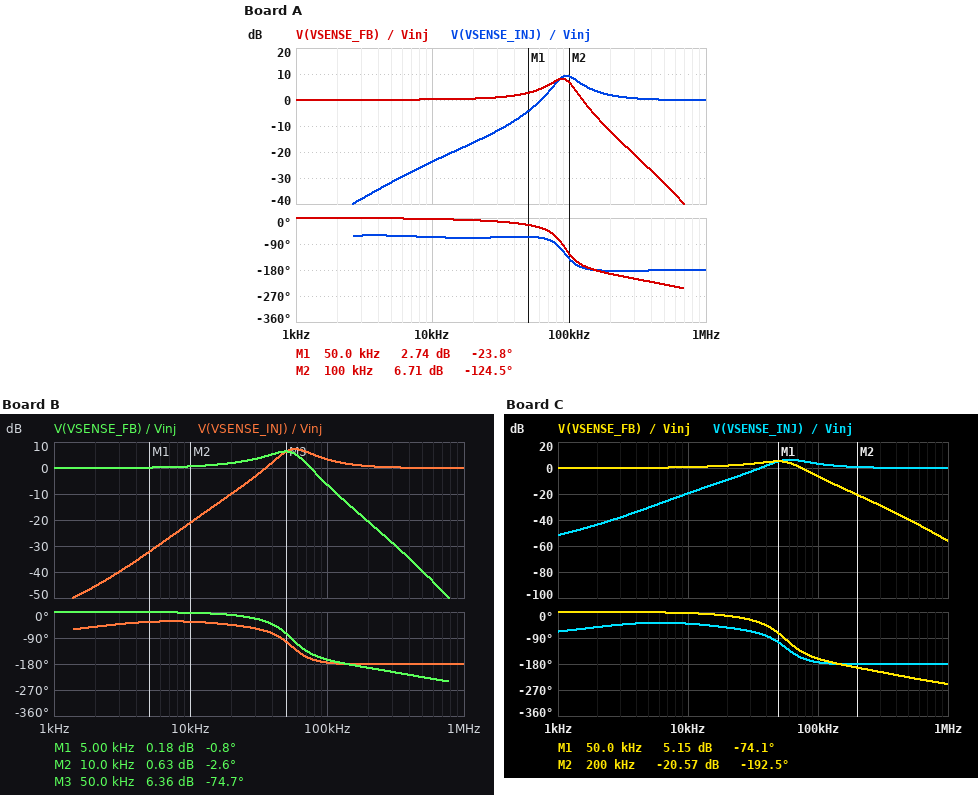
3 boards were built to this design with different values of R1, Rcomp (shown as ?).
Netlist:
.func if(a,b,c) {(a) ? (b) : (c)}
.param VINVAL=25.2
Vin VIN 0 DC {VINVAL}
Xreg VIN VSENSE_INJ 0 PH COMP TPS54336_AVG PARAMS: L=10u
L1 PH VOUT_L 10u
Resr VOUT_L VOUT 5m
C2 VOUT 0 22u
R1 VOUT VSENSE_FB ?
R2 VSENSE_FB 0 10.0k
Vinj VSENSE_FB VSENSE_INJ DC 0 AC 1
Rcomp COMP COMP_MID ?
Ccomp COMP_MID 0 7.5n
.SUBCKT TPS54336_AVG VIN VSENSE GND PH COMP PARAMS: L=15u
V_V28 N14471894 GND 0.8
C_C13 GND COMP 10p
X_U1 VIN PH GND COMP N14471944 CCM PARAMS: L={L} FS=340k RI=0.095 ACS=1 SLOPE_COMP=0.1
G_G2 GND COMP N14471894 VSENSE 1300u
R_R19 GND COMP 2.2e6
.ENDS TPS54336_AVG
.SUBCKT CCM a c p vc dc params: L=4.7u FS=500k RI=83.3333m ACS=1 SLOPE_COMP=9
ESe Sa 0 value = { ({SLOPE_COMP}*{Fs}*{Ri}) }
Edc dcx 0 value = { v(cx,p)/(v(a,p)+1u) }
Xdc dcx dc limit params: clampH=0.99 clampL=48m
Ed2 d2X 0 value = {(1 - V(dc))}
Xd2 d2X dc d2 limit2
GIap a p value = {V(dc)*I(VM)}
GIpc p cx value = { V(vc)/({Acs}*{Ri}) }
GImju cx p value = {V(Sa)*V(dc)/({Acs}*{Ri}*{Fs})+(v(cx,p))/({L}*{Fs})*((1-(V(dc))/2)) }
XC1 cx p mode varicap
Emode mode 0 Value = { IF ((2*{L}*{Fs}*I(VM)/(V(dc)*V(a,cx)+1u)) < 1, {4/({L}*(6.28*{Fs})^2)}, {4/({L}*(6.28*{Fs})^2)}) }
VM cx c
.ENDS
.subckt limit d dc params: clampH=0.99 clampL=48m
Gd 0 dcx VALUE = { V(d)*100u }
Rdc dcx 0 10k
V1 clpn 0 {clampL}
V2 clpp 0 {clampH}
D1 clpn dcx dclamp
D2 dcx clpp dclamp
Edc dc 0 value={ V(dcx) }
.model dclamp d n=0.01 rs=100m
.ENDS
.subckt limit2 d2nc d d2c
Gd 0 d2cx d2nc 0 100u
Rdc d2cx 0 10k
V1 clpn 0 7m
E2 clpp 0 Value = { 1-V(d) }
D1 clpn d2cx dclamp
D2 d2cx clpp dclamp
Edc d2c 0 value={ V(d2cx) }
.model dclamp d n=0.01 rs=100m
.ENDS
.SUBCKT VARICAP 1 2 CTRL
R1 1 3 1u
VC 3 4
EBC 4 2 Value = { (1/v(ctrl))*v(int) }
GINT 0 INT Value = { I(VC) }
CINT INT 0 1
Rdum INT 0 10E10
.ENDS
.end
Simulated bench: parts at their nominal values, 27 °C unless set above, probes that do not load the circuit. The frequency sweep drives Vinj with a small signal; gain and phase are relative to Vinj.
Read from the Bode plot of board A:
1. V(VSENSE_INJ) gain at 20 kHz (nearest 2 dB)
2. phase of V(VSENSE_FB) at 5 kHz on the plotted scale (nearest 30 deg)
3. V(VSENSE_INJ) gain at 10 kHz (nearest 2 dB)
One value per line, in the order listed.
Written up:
-16 dB
0 deg
-24 dB
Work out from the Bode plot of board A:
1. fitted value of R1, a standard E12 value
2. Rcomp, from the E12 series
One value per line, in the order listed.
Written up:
18 kΩ
3.9 kΩ
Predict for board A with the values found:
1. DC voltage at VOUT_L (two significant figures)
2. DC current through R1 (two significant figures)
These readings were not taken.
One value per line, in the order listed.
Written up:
2.2 V
80 µA
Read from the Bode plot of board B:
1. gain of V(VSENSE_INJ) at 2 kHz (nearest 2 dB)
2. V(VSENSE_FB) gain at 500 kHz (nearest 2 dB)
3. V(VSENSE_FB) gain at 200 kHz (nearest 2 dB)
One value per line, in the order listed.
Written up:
-46 dB
-40 dB
-20 dB
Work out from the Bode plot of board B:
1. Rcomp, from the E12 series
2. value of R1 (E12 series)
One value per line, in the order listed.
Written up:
1.2 kΩ
10 kΩ
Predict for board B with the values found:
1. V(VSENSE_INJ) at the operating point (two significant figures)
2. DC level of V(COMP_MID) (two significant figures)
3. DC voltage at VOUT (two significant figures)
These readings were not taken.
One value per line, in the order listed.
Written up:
800 mV
44 mV
1.6 V
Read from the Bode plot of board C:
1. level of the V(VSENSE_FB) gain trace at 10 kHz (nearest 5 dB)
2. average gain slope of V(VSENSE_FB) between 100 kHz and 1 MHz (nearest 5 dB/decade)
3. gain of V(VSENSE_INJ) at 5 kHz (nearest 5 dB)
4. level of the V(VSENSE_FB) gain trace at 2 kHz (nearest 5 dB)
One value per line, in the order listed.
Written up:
0 dB
-50 dB/decade
-30 dB
0 dB
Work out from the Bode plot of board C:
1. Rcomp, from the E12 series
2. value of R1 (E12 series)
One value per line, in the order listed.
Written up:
1.5 kΩ
15 kΩ
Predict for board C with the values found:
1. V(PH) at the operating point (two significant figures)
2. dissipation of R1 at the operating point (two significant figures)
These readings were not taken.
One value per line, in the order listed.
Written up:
2.0 V
96 µW
